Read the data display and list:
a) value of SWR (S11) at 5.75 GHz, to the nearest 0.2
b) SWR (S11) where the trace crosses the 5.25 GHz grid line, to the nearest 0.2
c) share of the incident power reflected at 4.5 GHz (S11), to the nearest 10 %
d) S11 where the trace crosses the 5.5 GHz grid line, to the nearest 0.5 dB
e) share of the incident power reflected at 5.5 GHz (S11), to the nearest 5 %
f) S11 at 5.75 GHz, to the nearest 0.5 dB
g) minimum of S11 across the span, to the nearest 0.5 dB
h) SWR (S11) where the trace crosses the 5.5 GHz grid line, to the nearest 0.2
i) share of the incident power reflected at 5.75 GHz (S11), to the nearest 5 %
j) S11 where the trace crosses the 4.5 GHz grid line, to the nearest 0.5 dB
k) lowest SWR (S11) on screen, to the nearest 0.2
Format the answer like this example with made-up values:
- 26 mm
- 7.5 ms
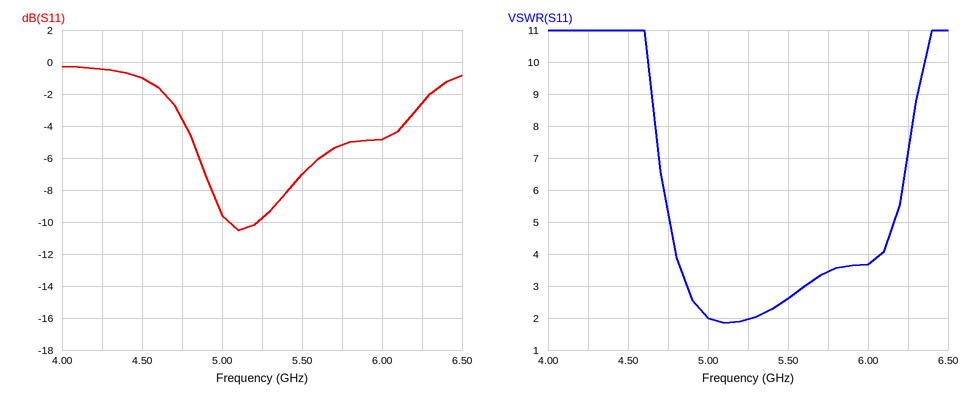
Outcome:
- 3.4
- 2.0
- 80 %
- -7.0 dB
- 20 %
- -5.0 dB
- -10.5 dB
- 2.6
- 30 %
- -1.0 dB
- 1.8
